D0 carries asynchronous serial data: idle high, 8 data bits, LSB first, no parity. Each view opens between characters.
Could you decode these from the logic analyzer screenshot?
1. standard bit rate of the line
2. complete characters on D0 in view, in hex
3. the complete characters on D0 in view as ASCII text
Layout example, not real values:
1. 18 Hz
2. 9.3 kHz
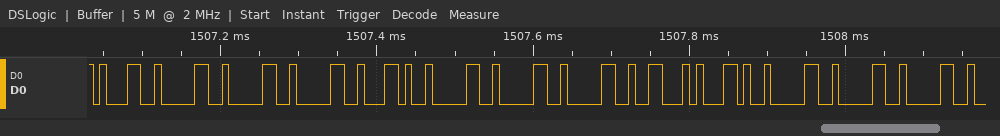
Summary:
1. 115200 baud
2. 31, 30, 30, 30, 2C, 30, 30, 30, 46, 2C, 30, 30, 30
3. "1000,000F,000"
